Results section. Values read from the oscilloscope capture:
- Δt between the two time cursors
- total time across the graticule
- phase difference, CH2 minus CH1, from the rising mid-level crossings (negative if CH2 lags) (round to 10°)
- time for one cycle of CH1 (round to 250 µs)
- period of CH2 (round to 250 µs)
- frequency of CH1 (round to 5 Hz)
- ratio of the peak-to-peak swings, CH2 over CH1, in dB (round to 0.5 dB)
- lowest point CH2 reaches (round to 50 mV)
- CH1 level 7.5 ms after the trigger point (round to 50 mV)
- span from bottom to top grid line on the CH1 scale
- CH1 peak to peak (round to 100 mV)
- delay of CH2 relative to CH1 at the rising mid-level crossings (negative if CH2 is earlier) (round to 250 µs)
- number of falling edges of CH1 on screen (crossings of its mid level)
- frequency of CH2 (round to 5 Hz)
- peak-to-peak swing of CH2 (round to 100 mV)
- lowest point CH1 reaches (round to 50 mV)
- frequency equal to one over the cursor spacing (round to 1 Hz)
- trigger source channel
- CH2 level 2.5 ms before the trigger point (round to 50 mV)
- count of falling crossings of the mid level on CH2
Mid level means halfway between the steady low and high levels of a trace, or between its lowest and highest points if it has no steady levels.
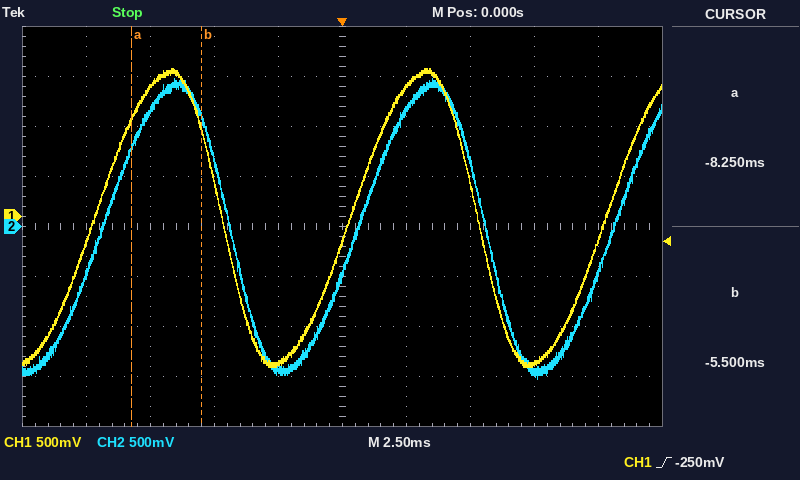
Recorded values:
2.75 ms
25 ms
-10°
10.00 ms
10.00 ms
100 Hz
0.0 dB
-1.50 V
-1.45 V
4 V
3.00 V
+250 µs
2
100 Hz
3.00 V
-1.50 V
364 Hz
CH1
-1.45 V
2
